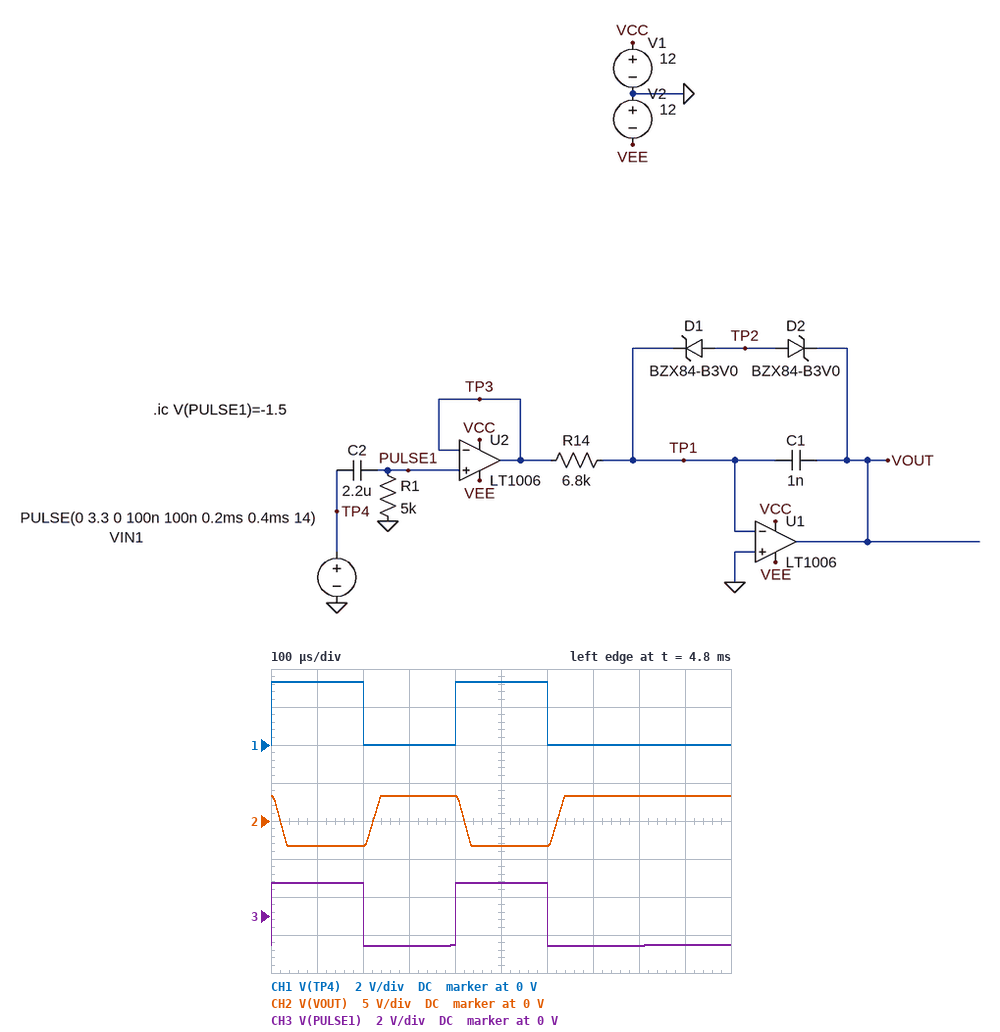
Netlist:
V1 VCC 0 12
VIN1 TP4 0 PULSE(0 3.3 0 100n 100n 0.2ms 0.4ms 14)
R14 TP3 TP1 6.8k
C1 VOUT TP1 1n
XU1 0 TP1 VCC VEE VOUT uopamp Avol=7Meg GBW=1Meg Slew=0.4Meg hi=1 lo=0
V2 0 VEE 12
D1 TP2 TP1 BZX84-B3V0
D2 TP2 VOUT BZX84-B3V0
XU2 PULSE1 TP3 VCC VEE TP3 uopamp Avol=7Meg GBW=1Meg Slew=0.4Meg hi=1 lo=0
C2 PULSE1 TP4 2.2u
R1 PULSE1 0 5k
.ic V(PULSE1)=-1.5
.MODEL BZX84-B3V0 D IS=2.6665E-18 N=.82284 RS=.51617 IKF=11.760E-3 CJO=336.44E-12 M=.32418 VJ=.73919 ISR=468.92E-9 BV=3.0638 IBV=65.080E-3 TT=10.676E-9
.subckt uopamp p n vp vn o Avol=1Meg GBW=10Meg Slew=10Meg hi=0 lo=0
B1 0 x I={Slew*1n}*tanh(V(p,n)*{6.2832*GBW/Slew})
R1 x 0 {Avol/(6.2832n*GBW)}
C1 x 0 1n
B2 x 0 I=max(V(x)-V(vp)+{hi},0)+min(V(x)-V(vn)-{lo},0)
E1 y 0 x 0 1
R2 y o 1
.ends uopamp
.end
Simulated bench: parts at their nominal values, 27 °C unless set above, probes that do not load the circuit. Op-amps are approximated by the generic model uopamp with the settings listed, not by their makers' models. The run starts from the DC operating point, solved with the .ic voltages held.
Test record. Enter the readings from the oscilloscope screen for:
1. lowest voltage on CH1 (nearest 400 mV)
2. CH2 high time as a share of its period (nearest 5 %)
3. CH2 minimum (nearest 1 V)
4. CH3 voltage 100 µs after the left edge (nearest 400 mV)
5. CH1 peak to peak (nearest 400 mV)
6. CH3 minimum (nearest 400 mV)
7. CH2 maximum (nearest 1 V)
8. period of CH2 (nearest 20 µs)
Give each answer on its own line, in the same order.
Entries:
0 V
50 %
-3 V
1.6 V
3.2 V
-1.6 V
3 V
400 µs
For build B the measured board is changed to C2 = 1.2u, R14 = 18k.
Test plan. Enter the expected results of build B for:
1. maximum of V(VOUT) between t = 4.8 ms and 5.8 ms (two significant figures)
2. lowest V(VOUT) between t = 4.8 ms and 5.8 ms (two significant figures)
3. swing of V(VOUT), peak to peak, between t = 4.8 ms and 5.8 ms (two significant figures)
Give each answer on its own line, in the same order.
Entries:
3.2 V
-3.2 V
6.4 V
